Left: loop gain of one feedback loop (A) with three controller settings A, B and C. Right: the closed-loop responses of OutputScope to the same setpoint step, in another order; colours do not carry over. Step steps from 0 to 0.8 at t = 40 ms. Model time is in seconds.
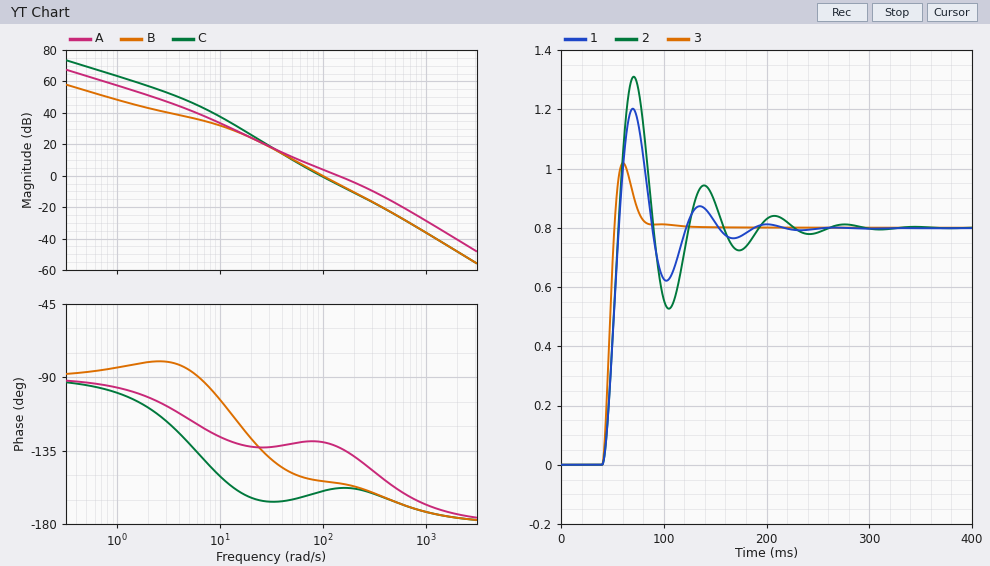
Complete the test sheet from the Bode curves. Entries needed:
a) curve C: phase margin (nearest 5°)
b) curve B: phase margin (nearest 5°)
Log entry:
20°
25°
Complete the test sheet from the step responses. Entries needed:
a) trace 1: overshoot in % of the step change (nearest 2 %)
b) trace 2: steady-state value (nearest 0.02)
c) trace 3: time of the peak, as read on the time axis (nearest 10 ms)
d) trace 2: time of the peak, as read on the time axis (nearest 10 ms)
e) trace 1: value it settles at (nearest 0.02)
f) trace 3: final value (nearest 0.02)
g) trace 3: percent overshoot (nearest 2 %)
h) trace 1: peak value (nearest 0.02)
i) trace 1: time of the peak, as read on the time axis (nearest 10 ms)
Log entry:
50 %
0.80
60 ms
70 ms
0.80
0.80
28 %
1.20
70 ms
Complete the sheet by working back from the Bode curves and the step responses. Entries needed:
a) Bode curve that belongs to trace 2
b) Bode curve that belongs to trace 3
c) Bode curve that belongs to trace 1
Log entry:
C
A
B
